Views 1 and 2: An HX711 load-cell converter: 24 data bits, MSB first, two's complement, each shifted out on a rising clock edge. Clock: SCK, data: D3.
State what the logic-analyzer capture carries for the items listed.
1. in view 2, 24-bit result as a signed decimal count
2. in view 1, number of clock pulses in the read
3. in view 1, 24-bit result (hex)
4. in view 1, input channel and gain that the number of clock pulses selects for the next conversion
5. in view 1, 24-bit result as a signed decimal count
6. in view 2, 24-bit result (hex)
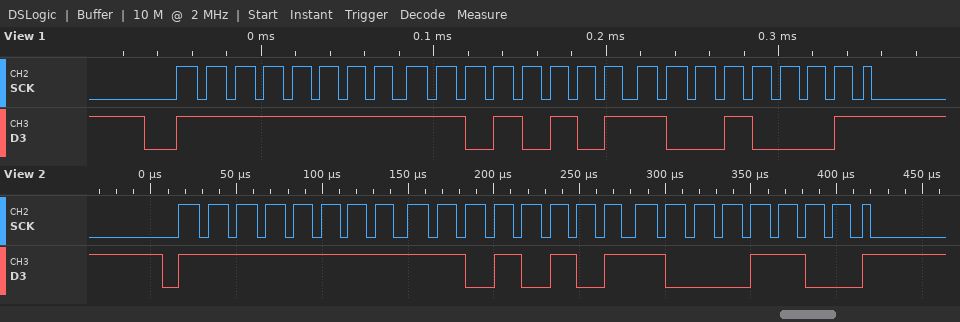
-10868
25
0xFFD591
channel A, gain 128
-10863
0xFFD58C
